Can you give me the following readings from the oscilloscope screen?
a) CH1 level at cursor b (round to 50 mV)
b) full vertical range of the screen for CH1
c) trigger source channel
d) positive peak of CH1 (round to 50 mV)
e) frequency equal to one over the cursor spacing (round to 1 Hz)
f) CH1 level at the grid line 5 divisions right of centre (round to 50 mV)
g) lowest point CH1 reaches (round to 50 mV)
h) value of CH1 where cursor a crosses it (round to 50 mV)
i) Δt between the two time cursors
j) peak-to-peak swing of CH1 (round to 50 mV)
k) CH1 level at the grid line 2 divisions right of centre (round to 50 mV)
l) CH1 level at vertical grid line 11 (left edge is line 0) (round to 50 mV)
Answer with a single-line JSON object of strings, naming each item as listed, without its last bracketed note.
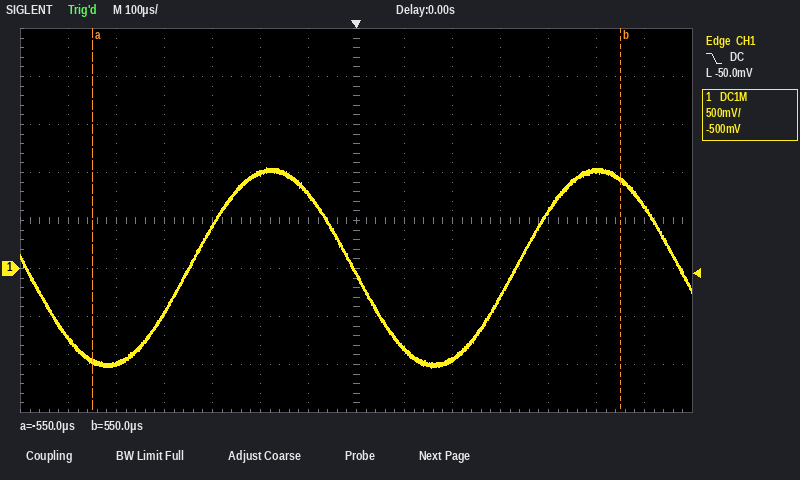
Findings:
{"CH1 level at cursor b": "900 mV", "full vertical range of the screen for CH1": "4 V", "trigger source channel": "CH1", "positive peak of CH1": "1.05 V", "frequency equal to one over the cursor spacing": "909 Hz", "CH1 level at the grid line 5 divisions right of centre": "1.00 V", "lowest point CH1 reaches": "-1.05 V", "value of CH1 where cursor a crosses it": "-950 mV", "Δt between the two time cursors": "1.10 ms", "peak-to-peak swing of CH1": "2.10 V", "CH1 level at the grid line 2 divisions right of centre": "-950 mV", "CH1 level at vertical grid line 11 (left edge is line 0)": "600 mV"}
